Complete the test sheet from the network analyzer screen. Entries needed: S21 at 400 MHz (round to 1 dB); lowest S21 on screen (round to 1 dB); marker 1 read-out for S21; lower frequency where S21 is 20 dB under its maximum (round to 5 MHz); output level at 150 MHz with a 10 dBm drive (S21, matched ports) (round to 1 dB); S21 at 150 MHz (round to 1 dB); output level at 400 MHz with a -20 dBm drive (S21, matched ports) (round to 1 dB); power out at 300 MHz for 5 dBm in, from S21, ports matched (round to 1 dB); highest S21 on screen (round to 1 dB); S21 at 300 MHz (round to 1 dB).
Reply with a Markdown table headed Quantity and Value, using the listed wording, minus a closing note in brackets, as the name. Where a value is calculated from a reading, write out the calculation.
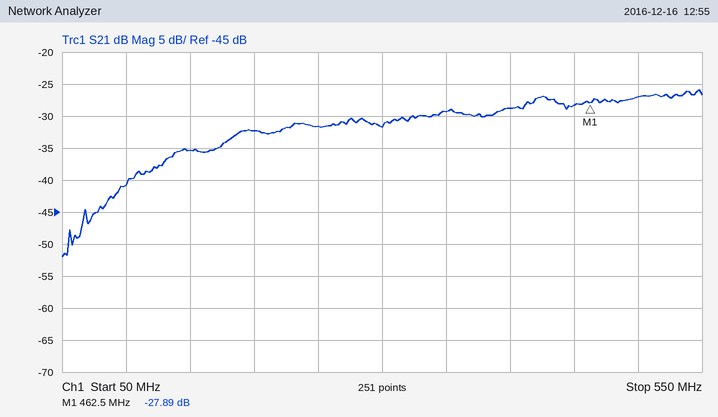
| Quantity | Value |
|---|---|
| S21 at 400 MHz | -29 dB |
| lowest S21 on screen | -52 dB |
| marker 1 read-out for S21 | -27.89 dB |
| lower frequency where S21 is 20 dB under its maximum | 75 MHz |
| output level at 150 MHz with a 10 dBm drive (S21, matched ports) | 10 dBm + (-35 dB) = -25 dBm |
| S21 at 150 MHz | -35 dB |
| output level at 400 MHz with a -20 dBm drive (S21, matched ports) | -20 dBm + (-29 dB) = -49 dBm |
| power out at 300 MHz for 5 dBm in, from S21, ports matched | 5 dBm + (-32 dB) = -27 dBm |
| highest S21 on screen | -26 dB |
| S21 at 300 MHz | -32 dB |
